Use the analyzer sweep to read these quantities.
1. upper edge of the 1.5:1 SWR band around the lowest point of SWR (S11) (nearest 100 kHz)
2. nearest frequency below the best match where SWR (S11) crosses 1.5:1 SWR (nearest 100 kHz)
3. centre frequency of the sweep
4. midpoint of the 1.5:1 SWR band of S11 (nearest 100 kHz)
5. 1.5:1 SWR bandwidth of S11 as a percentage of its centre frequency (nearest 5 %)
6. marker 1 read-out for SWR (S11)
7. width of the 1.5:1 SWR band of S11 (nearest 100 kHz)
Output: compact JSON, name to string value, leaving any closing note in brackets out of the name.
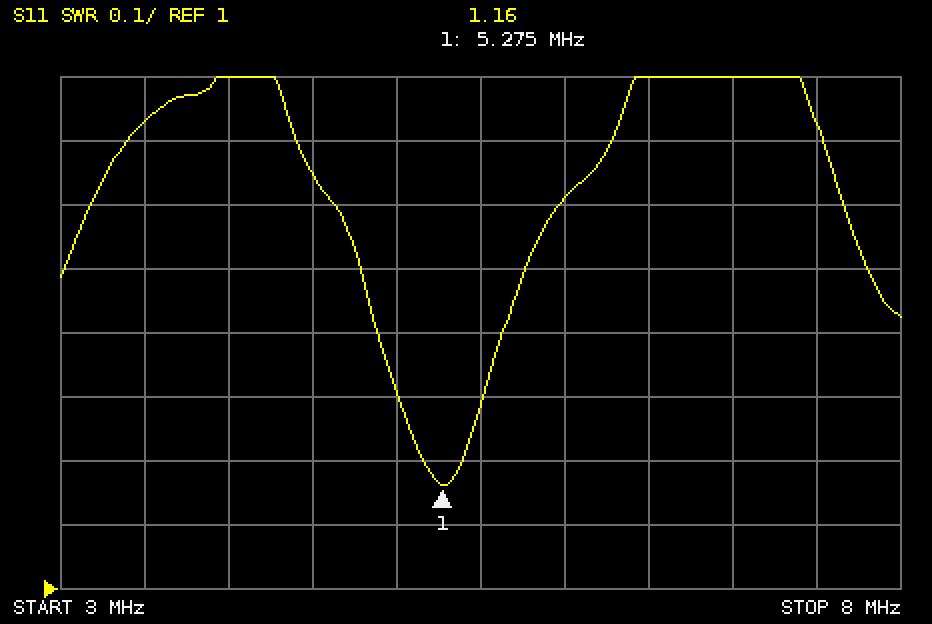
{"upper edge of the 1.5:1 SWR band around the lowest point of SWR (S11)": "5.8 MHz", "nearest frequency below the best match where SWR (S11) crosses 1.5:1 SWR": "4.8 MHz", "centre frequency of the sweep": "5.5 MHz", "midpoint of the 1.5:1 SWR band of S11": "5.3 MHz", "1.5:1 SWR bandwidth of S11 as a percentage of its centre frequency": "20 %", "marker 1 read-out for SWR": "1.16", "width of the 1.5:1 SWR band of S11": "1.0 MHz"}
